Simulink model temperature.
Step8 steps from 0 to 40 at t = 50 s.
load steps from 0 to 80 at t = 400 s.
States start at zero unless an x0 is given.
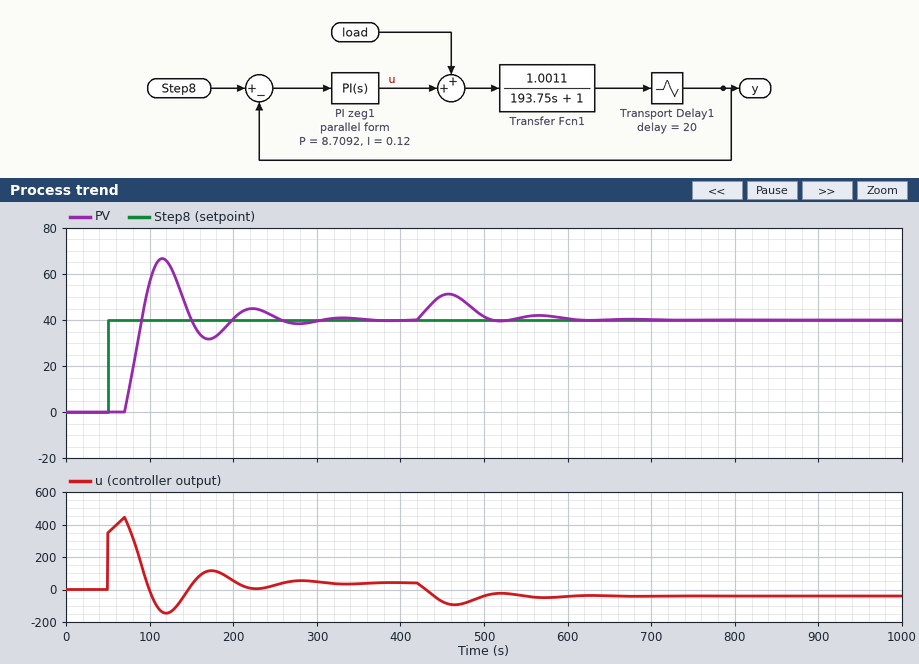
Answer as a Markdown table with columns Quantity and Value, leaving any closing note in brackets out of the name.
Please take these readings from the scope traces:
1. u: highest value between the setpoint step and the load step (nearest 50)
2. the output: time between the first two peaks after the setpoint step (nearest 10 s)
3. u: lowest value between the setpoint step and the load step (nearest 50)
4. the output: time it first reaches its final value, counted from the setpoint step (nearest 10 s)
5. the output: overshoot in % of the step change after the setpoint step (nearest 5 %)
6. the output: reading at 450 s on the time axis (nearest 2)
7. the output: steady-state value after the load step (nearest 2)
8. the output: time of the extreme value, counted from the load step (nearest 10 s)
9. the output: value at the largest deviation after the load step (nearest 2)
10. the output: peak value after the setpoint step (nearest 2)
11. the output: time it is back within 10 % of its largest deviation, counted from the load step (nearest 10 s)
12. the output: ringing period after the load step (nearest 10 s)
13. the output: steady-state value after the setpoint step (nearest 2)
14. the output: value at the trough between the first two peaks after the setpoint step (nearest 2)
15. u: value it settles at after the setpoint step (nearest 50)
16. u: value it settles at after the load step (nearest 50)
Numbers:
| Quantity | Value |
|---|---|
| u: highest value between the setpoint step and the load step | 450 |
| the output: time between the first two peaks after the setpoint step | 110 s |
| u: lowest value between the setpoint step and the load step | -150 |
| the output: time it first reaches its final value, counted from the setpoint step | 40 s |
| the output: overshoot in % of the step change after the setpoint step | 65 % |
| the output: reading at 450 s on the time axis | 50 |
| the output: steady-state value after the load step | 40 |
| the output: time of the extreme value, counted from the load step | 60 s |
| the output: value at the largest deviation after the load step | 52 |
| the output: peak value after the setpoint step | 66 |
| the output: time it is back within 10 % of its largest deviation, counted from the load step | 190 s |
| the output: ringing period after the load step | 110 s |
| the output: steady-state value after the setpoint step | 40 |
| the output: value at the trough between the first two peaks after the setpoint step | 32 |
| u: value it settles at after the setpoint step | 50 |
| u: value it settles at after the load step | -50 |
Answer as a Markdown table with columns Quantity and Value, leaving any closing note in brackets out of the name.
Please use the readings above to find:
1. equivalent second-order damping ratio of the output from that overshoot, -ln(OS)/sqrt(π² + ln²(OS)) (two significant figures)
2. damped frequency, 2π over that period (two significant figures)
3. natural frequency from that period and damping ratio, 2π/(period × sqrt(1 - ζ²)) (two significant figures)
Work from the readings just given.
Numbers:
| Quantity | Value |
|---|---|
| equivalent second-order damping ratio of the output from that overshoot, -ln(OS)/sqrt(π² + ln²(OS)) | 0.14 |
| damped frequency, 2π over that period | 0.057 rad/s |
| natural frequency from that period and damping ratio, 2π/(period × sqrt(1 - ζ²)) | 0.058 rad/s |
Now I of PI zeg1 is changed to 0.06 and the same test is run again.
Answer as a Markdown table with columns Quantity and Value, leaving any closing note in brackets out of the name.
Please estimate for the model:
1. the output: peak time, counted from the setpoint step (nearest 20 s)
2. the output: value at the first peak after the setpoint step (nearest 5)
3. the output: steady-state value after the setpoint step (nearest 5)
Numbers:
| Quantity | Value |
|---|---|
| the output: peak time, counted from the setpoint step | 60 s |
| the output: value at the first peak after the setpoint step | 60 |
| the output: steady-state value after the setpoint step | 40 |
